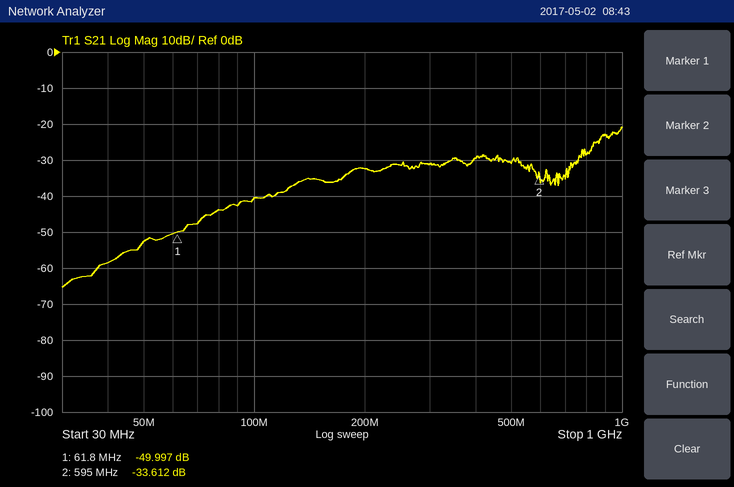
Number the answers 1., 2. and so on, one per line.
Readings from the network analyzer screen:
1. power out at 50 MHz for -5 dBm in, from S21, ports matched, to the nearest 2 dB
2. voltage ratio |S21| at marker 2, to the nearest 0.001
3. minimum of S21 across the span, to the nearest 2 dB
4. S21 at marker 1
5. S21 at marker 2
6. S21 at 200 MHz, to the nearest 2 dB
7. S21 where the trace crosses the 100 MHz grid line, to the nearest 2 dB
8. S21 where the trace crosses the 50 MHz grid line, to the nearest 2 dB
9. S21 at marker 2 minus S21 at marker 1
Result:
1. -58 dBm
2. 0.021
3. -66 dB
4. -49.997 dB
5. -33.612 dB
6. -32 dB
7. -40 dB
8. -52 dB
9. 16.385 dB
